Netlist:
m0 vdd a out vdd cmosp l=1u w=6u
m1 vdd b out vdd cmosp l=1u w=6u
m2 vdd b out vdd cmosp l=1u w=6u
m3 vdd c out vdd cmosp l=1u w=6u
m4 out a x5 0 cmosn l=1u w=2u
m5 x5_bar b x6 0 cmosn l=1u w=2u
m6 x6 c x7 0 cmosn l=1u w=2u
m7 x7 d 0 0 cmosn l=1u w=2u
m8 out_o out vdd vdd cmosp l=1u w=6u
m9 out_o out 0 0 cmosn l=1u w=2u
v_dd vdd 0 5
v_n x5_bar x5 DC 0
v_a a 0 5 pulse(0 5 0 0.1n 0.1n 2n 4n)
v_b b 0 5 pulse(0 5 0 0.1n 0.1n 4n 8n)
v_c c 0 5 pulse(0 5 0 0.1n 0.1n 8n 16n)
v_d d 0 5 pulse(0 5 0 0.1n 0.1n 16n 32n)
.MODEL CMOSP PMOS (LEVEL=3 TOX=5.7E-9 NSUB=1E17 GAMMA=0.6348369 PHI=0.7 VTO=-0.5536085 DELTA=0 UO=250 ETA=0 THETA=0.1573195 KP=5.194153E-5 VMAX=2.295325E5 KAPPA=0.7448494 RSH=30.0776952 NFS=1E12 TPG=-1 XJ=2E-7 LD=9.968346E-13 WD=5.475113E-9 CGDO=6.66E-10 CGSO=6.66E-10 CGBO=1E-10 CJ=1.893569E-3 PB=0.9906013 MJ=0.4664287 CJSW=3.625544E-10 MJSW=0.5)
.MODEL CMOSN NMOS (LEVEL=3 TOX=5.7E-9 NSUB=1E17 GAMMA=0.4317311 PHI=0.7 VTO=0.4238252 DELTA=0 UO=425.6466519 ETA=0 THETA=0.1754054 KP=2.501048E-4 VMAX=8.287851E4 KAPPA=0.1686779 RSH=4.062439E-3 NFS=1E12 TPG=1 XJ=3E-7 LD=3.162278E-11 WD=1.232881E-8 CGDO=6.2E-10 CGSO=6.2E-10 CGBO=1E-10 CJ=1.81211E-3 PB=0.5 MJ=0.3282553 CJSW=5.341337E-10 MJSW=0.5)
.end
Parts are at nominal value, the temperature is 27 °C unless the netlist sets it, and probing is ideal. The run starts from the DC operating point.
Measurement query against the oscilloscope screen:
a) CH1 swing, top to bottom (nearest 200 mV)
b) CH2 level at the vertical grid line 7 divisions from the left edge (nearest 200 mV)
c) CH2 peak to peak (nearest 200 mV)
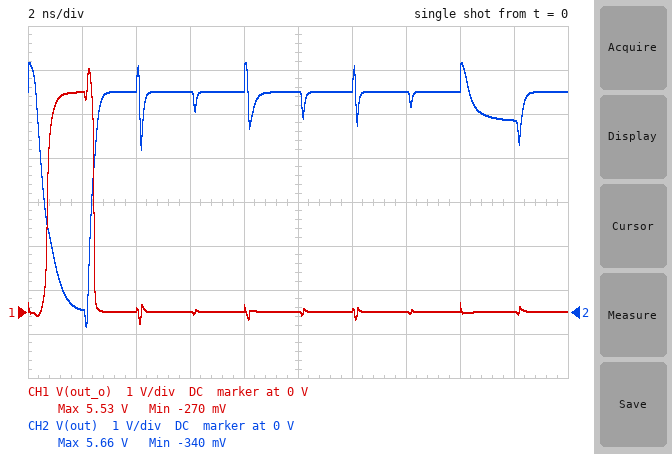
5.8 V
5.0 V
6.0 V
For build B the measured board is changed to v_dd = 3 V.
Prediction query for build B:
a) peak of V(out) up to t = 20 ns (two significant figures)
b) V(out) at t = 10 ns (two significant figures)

3.7 V
3.0 V
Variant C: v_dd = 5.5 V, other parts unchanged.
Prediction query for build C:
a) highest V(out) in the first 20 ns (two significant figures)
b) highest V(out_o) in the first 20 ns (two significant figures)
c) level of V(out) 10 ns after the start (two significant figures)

6.2 V
6.1 V
5.5 V
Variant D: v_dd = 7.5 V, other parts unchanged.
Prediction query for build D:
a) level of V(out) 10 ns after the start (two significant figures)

7.5 V
